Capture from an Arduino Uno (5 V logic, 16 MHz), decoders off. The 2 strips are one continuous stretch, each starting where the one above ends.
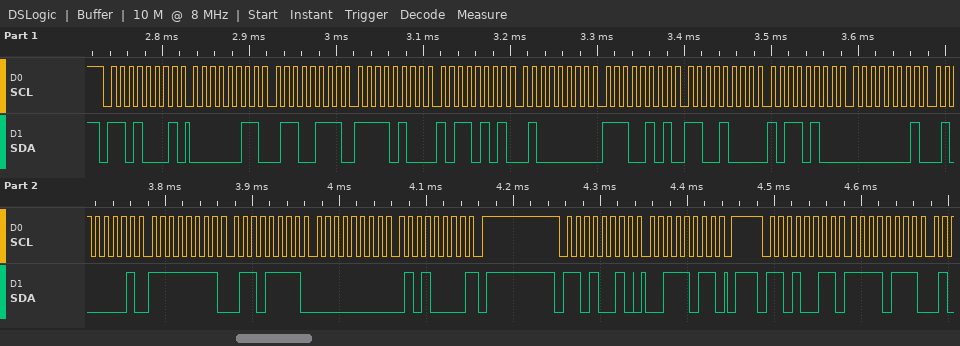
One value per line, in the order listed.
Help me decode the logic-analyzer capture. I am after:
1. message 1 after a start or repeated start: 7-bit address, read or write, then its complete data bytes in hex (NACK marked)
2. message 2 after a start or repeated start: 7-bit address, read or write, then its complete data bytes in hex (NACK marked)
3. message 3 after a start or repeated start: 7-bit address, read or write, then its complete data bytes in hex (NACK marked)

0x68 read: 03 67 F4 B5 40 E5 C8 B4 01 41 FF 6F 00 50 NACK
0x69 write: 3B
0x69 read: F7
